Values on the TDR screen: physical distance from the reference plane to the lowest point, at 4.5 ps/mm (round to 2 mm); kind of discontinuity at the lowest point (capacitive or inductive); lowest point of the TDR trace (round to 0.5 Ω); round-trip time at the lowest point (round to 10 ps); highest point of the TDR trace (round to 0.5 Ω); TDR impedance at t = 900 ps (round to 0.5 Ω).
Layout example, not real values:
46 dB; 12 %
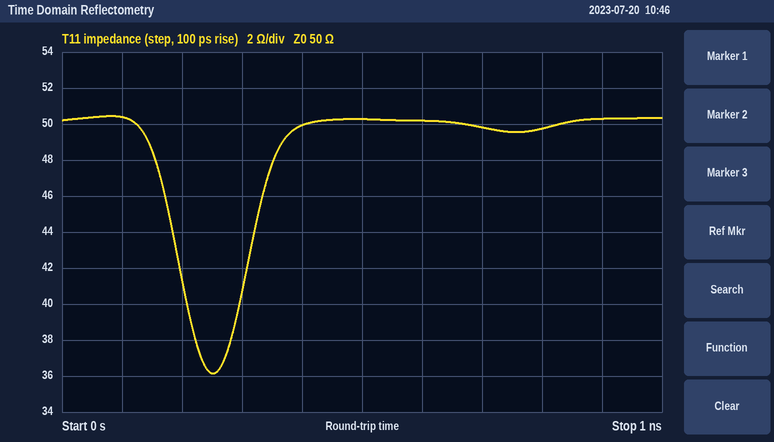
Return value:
28 mm; capacitive; 36.0 Ω; 250 ps; 50.5 Ω; 50.5 Ω
